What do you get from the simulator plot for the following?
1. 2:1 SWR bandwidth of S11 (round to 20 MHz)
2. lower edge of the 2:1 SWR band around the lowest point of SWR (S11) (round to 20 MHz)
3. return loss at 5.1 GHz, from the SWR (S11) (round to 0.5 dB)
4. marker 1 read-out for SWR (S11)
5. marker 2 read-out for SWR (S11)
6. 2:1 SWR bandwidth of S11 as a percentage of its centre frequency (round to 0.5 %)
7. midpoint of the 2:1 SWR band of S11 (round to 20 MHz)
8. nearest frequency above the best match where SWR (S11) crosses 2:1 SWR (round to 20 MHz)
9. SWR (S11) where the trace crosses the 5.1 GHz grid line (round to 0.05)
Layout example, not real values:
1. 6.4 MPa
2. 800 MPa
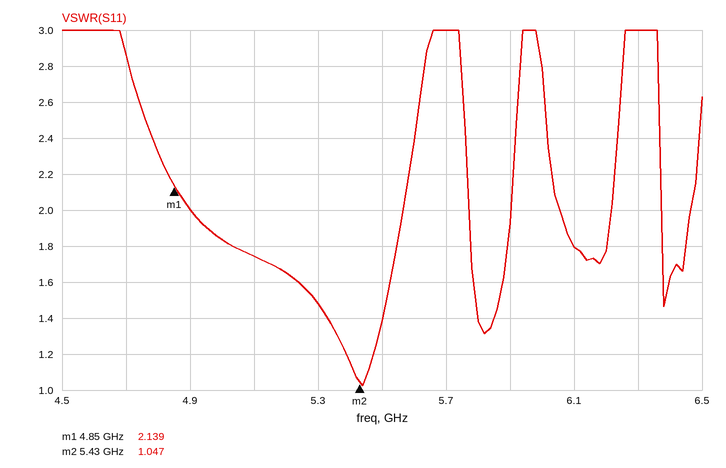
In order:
1. 660 MHz
2. 4.90 GHz
3. 11.5 dB
4. 2.139
5. 1.047
6. 12.5 %
7. 5.24 GHz
8. 5.56 GHz
9. 1.75
